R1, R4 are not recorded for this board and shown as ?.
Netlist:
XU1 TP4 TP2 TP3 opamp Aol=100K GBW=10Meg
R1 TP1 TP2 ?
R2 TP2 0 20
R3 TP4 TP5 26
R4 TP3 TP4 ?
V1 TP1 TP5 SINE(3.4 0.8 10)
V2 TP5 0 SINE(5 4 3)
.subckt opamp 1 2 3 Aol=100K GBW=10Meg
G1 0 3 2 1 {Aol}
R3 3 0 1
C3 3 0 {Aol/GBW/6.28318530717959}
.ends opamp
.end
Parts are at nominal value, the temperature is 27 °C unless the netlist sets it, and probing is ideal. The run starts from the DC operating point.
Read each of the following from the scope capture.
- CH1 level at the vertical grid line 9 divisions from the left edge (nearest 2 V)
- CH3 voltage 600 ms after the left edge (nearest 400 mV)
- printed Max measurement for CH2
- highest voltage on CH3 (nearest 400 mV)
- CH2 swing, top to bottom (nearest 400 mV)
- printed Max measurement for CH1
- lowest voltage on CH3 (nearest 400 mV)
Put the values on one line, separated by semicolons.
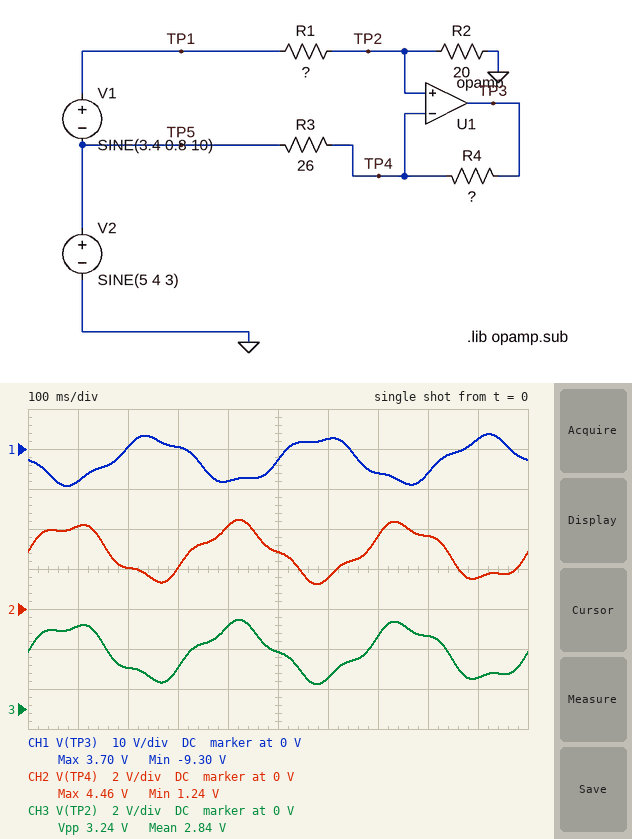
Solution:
2 V; 1.6 V; 4.46 V; 4.4 V; 3.2 V; 3.70 V; 1.2 V
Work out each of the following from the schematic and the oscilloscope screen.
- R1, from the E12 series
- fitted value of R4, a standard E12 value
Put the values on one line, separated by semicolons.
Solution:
39 Ω; 68 Ω
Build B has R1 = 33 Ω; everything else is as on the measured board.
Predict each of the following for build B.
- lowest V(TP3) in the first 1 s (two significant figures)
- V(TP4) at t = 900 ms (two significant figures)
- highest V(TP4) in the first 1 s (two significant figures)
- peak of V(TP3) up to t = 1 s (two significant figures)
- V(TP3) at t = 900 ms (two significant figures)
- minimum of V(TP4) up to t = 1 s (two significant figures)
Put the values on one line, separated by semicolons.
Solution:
-7.7 V; 1.7 V; 5.0 V; 4.4 V; 3.1 V; 1.4 V
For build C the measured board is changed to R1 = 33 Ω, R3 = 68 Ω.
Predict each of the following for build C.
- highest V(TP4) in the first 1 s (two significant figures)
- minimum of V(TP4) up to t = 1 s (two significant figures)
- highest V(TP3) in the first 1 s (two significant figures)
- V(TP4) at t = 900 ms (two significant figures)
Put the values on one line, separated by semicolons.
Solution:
5.0 V; 1.4 V; 2.9 V; 1.7 V
